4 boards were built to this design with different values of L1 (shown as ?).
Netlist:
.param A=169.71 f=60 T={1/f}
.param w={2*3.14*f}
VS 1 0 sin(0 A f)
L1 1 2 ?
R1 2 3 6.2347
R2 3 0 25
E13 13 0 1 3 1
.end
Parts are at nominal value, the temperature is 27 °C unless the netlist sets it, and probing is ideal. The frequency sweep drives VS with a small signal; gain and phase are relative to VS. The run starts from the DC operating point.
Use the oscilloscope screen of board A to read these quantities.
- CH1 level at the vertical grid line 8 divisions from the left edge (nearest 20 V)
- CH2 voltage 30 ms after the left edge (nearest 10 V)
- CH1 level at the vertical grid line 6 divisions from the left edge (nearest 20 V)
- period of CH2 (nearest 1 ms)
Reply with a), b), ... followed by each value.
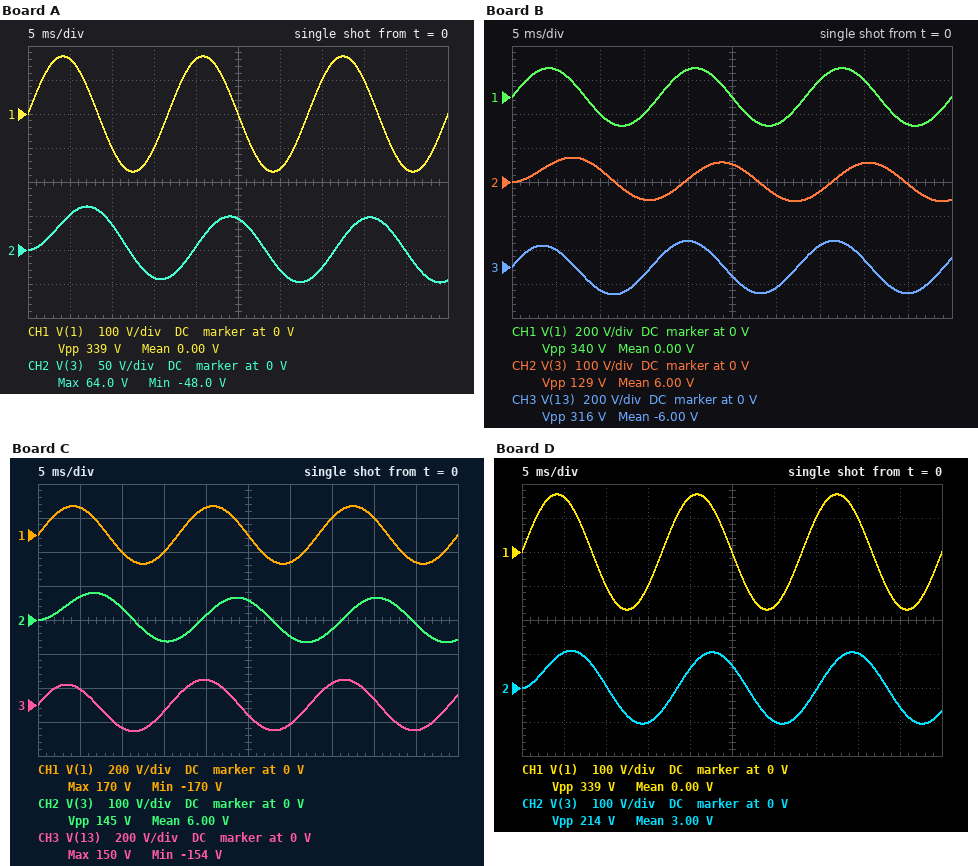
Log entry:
a) 100 V
b) -30 V
c) -160 V
d) 17 ms
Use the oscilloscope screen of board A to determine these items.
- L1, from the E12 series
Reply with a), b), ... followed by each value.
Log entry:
a) 220 mH
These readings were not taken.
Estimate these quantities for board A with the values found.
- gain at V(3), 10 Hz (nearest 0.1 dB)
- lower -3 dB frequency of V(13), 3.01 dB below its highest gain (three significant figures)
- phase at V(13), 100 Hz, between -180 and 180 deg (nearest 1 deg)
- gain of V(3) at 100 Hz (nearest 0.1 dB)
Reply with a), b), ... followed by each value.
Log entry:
a) -2.7 dB
b) 21.7 Hz
c) 10 deg
d) -15.1 dB
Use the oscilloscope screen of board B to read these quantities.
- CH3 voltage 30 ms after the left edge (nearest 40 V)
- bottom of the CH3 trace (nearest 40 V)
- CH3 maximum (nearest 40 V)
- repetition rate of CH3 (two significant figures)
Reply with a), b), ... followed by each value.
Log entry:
a) -120 V
b) -160 V
c) 160 V
d) 60 Hz
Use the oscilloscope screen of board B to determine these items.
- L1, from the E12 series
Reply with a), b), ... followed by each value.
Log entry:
a) 180 mH
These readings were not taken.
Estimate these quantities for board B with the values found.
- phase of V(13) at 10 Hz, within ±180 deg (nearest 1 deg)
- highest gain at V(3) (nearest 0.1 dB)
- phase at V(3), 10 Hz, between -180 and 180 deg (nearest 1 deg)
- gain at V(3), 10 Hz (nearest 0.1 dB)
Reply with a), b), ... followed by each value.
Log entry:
a) 41 deg
b) -1.9 dB
c) -20 deg
d) -2.5 dB
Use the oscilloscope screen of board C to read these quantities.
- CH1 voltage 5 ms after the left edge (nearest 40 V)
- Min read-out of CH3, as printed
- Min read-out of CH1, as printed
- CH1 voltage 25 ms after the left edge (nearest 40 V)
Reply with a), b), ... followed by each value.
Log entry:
a) 160 V
b) -154 V
c) -170 V
d) 0 V
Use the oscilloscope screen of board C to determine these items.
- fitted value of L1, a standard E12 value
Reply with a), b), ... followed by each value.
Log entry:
a) 150 mH
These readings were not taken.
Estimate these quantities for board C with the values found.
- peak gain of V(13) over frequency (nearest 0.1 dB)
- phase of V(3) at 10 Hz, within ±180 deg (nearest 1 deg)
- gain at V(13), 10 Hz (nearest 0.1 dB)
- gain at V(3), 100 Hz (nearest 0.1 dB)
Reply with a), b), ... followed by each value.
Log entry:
a) 0 dB
b) -17 deg
c) -9.2 dB
d) -12.0 dB
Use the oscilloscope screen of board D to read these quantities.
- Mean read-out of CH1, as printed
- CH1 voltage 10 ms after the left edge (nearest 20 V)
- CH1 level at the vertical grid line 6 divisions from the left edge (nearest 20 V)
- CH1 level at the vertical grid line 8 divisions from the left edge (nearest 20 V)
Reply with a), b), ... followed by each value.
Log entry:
a) 0.00 V
b) -100 V
c) -160 V
d) 100 V
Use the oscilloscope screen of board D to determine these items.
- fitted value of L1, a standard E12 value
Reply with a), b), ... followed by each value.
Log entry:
a) 68 mH
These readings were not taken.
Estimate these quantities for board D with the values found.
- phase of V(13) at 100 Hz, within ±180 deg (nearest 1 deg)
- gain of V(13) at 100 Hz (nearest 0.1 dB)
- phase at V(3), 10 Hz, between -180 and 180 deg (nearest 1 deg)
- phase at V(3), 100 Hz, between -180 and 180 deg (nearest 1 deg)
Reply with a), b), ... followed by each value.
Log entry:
a) 28 deg
b) -1.8 dB
c) -8 deg
d) -54 deg
